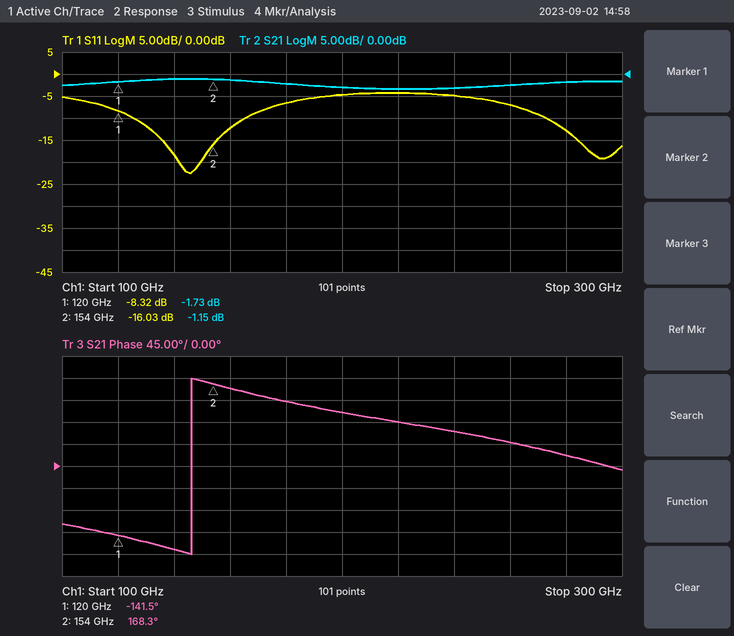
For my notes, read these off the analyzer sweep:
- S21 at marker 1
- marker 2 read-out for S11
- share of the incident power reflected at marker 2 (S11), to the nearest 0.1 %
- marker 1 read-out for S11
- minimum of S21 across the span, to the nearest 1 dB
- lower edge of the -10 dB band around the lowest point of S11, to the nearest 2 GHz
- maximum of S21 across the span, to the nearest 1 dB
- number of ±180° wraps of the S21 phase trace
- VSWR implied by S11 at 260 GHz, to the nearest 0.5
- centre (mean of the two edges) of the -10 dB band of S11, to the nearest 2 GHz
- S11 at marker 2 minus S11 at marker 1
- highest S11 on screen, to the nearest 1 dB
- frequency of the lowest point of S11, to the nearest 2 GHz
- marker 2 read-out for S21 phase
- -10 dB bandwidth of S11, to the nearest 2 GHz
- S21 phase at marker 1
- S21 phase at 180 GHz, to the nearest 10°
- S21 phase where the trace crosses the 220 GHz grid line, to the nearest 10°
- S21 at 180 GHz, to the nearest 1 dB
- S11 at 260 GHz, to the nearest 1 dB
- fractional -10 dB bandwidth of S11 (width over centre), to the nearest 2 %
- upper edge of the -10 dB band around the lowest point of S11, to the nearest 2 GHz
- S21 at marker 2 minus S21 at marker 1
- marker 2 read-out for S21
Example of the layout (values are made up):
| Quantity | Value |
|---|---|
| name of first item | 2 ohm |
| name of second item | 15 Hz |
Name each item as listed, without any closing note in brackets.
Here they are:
| Quantity | Value |
|---|---|
| S21 at marker 1 | -1.73 dB |
| marker 2 read-out for S11 | -16.03 dB |
| share of the incident power reflected at marker 2 (S11), to the nearest 0.1 % | 2.5 % |
| marker 1 read-out for S11 | -8.32 dB |
| minimum of S21 across the span, to the nearest 1 dB | -3 dB |
| lower edge of the -10 dB band around the lowest point of S11, to the nearest 2 GHz | 126 GHz |
| maximum of S21 across the span, to the nearest 1 dB | -1 dB |
| number of ±180° wraps of the S21 phase trace | 1 |
| VSWR implied by S11 at 260 GHz, to the nearest 0.5 | 2.5 |
| centre (mean of the two edges) of the -10 dB band of S11, to the nearest 2 GHz | 146 GHz |
| S11 at marker 2 minus S11 at marker 1 | -7.71 dB |
| highest S11 on screen, to the nearest 1 dB | -4 dB |
| frequency of the lowest point of S11, to the nearest 2 GHz | 146 GHz |
| marker 2 read-out for S21 phase | 168.3° |
| -10 dB bandwidth of S11, to the nearest 2 GHz | 40 GHz |
| S21 phase at marker 1 | -141.5° |
| S21 phase at 180 GHz, to the nearest 10° | 130° |
| S21 phase where the trace crosses the 220 GHz grid line, to the nearest 10° | 90° |
| S21 at 180 GHz, to the nearest 1 dB | -2 dB |
| S11 at 260 GHz, to the nearest 1 dB | -7 dB |
| fractional -10 dB bandwidth of S11 (width over centre), to the nearest 2 % | 28 % |
| upper edge of the -10 dB band around the lowest point of S11, to the nearest 2 GHz | 166 GHz |
| S21 at marker 2 minus S21 at marker 1 | 0.58 dB |
| marker 2 read-out for S21 | -1.15 dB |
